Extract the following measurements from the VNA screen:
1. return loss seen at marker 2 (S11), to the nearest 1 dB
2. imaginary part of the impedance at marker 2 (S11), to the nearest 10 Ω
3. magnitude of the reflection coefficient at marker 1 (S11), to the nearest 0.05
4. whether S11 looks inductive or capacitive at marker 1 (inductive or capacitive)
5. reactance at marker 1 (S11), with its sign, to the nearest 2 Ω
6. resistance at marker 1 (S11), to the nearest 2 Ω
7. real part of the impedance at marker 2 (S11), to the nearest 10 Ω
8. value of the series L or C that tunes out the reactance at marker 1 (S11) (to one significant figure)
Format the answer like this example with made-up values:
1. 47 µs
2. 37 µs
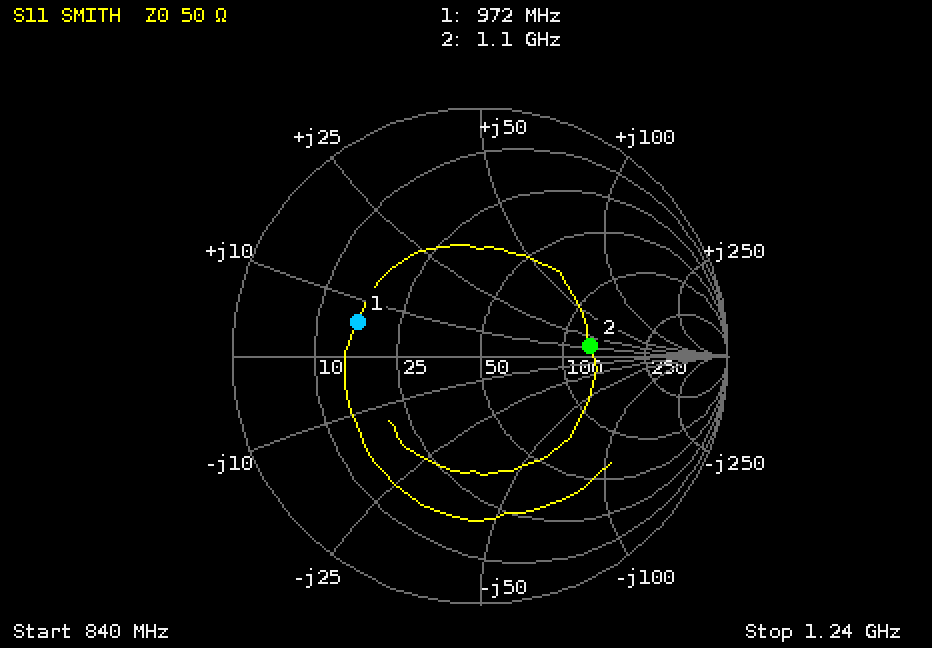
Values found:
1. 7 dB
2. +10 Ω
3. 0.50
4. inductive
5. +6 Ω
6. 16 Ω
7. 130 Ω
8. 30 pF
